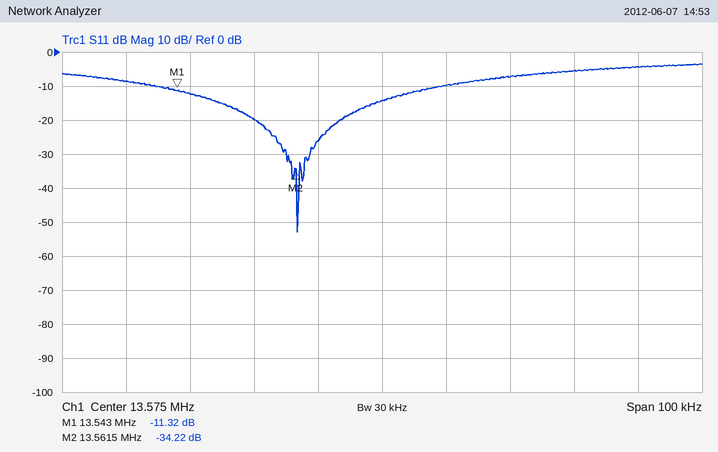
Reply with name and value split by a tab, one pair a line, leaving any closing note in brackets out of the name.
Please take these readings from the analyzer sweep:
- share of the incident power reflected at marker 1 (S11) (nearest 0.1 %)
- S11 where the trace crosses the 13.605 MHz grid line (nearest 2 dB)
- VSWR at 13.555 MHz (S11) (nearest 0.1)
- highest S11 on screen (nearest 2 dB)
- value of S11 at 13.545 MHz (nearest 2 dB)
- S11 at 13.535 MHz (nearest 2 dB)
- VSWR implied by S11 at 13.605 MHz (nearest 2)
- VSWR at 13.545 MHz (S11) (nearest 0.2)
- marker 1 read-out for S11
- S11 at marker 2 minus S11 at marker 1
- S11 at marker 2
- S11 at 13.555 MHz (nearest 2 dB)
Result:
share of the incident power reflected at marker 1 (S11)	7.4 %
S11 where the trace crosses the 13.605 MHz grid line	-6 dB
VSWR at 13.555 MHz (S11)	1.2
highest S11 on screen	-4 dB
value of S11 at 13.545 MHz	-12 dB
S11 at 13.535 MHz	-8 dB
VSWR implied by S11 at 13.605 MHz	4
VSWR at 13.545 MHz (S11)	1.6
marker 1 read-out for S11	-11.32 dB
S11 at marker 2 minus S11 at marker 1	-22.90 dB
S11 at marker 2	-34.22 dB
S11 at 13.555 MHz	-20 dB
